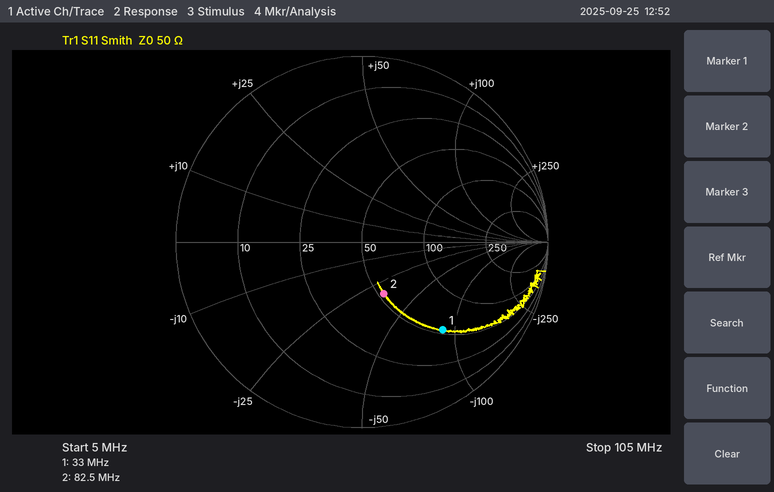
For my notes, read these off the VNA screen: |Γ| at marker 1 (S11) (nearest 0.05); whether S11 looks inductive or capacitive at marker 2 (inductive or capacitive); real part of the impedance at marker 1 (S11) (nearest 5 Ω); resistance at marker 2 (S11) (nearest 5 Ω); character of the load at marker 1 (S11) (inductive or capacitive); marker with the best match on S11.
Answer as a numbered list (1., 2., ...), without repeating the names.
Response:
1. 0.65
2. capacitive
3. 55 Ω
4. 55 Ω
5. capacitive
6. marker 2
